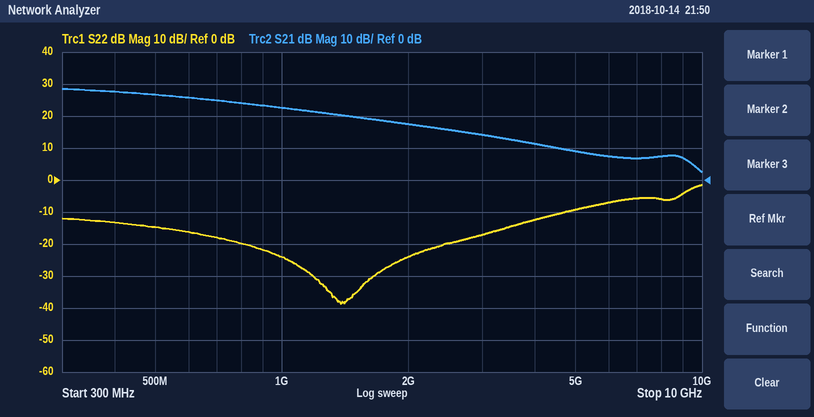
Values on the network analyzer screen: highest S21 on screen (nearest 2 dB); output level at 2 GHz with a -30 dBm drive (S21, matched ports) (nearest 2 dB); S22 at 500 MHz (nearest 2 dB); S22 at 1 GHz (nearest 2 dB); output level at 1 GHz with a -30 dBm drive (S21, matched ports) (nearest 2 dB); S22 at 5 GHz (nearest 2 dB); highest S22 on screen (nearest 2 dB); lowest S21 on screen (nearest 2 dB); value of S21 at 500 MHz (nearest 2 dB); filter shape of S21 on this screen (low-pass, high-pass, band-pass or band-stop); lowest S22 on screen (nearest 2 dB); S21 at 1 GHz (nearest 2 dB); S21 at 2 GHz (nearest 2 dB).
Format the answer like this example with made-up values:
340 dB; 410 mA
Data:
28 dB; -12 dBm; -14 dB; -24 dB; -8 dBm; -10 dB; -2 dB; 2 dB; 26 dB; low-pass; -38 dB; 22 dB; 18 dB
